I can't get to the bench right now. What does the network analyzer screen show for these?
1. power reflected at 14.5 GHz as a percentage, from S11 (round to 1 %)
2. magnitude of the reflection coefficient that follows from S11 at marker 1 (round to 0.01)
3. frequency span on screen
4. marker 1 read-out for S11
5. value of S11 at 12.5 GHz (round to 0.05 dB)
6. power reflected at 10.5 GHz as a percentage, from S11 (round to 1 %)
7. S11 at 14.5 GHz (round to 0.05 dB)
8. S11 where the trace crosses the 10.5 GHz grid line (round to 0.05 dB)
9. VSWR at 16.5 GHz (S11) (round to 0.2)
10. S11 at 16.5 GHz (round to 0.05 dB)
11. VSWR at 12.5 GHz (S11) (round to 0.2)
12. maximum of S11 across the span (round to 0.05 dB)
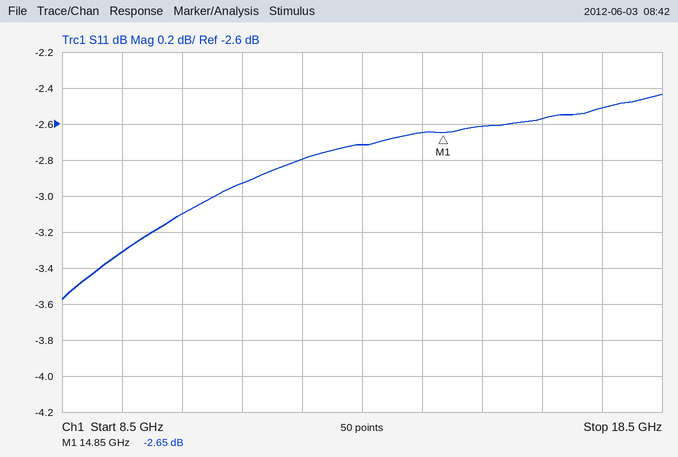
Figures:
54 %
0.74
10 GHz
-2.65 dB
-2.80 dB
49 %
-2.65 dB
-3.10 dB
6.8
-2.55 dB
6.2
-2.45 dB
